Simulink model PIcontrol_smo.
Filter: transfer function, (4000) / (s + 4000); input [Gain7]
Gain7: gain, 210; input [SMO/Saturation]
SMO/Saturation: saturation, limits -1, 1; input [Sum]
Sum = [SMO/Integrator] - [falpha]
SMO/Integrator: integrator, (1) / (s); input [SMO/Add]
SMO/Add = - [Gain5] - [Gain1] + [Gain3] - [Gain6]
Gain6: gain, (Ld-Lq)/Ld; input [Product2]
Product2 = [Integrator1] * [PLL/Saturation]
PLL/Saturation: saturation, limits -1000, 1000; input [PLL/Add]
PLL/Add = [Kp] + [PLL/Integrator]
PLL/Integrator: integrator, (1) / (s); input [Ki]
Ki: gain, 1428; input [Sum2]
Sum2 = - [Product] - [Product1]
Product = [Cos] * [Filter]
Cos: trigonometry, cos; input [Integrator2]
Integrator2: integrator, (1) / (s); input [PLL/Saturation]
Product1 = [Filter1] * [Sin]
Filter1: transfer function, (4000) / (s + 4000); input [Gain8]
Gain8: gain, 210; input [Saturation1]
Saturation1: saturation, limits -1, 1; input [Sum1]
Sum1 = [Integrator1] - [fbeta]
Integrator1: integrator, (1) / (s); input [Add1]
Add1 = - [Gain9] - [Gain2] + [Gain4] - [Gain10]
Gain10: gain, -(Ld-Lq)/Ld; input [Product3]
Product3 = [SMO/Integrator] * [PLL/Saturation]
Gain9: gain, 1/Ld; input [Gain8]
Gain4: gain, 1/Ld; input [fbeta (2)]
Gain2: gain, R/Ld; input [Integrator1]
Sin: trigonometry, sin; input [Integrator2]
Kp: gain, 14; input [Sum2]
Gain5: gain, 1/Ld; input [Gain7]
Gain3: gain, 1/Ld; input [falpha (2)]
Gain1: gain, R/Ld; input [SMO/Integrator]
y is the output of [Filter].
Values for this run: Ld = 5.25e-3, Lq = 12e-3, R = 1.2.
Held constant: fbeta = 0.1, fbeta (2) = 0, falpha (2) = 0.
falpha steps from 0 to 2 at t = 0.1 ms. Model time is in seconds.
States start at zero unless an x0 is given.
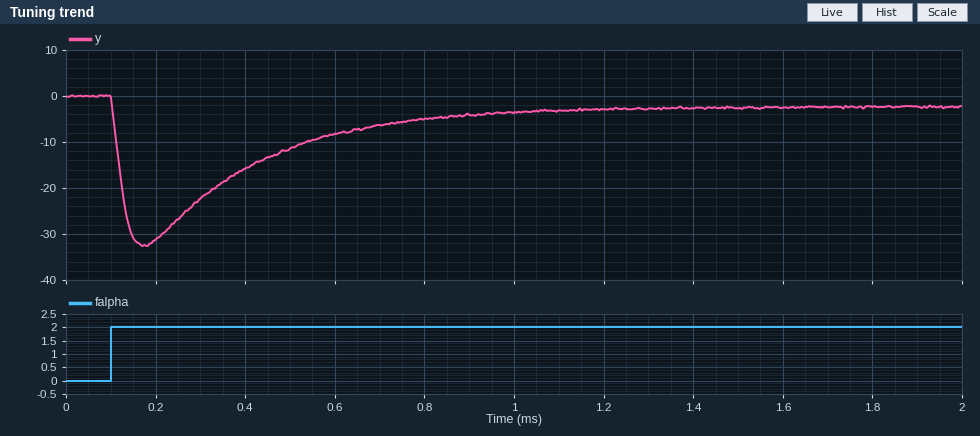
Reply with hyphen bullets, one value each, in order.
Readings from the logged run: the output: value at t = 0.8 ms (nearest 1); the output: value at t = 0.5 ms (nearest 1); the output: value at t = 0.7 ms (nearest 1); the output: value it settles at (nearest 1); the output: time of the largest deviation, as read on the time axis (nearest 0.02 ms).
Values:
- -5
- -11
- -6
- -2
- 0.18 ms
